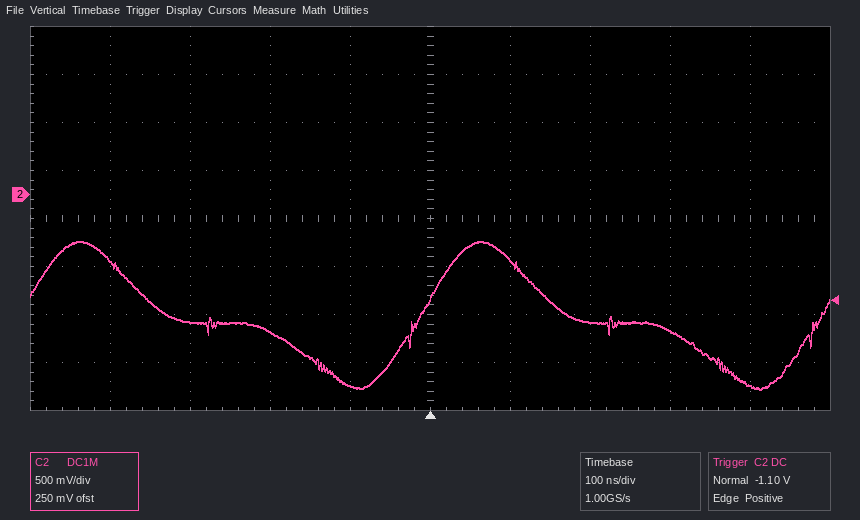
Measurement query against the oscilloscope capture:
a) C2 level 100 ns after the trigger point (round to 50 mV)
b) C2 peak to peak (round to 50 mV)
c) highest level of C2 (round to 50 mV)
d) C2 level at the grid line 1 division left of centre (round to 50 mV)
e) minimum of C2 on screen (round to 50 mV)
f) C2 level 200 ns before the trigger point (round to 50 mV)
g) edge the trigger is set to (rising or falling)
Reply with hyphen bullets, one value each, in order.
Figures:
- -700 mV
- 1.55 V
- -500 mV
- -2.00 V
- -2.05 V
- -1.45 V
- rising
